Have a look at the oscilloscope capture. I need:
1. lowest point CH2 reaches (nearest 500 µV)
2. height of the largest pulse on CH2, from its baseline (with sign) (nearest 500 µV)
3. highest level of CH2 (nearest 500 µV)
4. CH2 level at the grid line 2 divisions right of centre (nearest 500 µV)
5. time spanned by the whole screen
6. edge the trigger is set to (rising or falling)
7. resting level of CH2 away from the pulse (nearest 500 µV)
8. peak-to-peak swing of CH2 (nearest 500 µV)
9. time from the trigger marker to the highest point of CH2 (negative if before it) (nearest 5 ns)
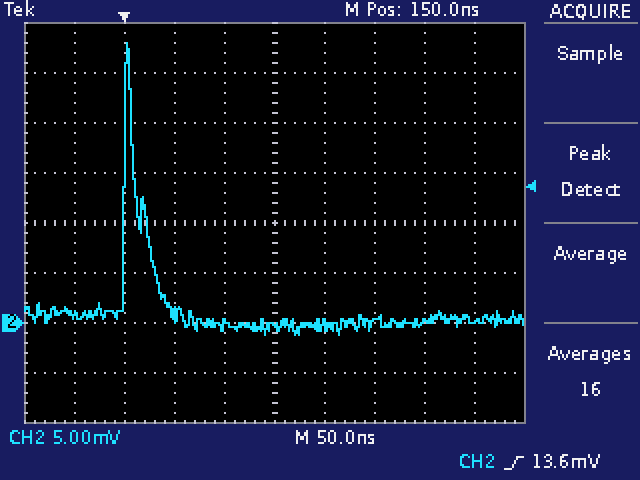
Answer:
-1.0 mV
+28.0 mV
28.0 mV
0.0 mV
500 ns
rising
0.0 mV
29.0 mV
+5 ns
